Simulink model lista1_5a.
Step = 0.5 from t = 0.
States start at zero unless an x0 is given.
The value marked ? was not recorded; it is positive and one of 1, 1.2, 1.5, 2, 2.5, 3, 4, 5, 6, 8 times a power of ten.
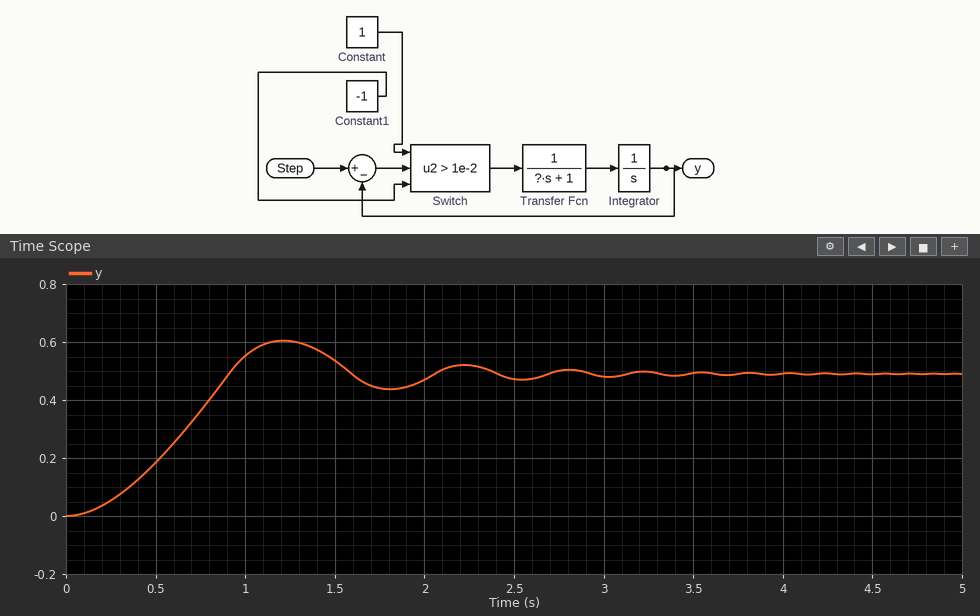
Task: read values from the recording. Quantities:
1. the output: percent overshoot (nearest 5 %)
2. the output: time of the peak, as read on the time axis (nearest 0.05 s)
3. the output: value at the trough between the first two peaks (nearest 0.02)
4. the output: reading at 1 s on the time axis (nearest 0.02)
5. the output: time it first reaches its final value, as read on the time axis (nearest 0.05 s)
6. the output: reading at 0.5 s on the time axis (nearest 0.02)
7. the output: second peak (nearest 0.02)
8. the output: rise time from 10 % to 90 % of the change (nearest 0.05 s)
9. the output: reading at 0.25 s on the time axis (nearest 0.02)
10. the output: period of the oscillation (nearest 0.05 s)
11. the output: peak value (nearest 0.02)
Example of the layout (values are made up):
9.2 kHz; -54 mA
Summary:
25 %; 1.20 s; 0.44; 0.56; 0.90 s; 0.18; 0.52; 0.60 s; 0.06; 1.00 s; 0.60
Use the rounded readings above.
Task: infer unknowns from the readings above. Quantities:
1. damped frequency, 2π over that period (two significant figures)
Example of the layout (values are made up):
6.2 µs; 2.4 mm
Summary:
6.3 rad/s
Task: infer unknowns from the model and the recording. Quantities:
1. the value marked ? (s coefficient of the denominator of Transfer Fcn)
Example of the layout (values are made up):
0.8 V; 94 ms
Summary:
0.5
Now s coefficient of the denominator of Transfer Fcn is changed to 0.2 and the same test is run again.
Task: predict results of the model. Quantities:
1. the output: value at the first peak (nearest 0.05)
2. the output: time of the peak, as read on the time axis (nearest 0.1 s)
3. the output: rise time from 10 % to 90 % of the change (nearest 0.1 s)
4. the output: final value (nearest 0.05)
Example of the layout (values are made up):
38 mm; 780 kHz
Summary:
0.55; 0.8 s; 0.5 s; 0.50
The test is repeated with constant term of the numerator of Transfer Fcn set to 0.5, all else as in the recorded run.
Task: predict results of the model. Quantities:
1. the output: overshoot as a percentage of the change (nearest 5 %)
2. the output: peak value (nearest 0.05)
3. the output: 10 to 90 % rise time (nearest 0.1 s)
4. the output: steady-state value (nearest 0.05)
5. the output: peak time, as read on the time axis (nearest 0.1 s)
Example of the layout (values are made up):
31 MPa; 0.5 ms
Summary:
15 %; 0.55; 1.0 s; 0.50; 1.8 s
